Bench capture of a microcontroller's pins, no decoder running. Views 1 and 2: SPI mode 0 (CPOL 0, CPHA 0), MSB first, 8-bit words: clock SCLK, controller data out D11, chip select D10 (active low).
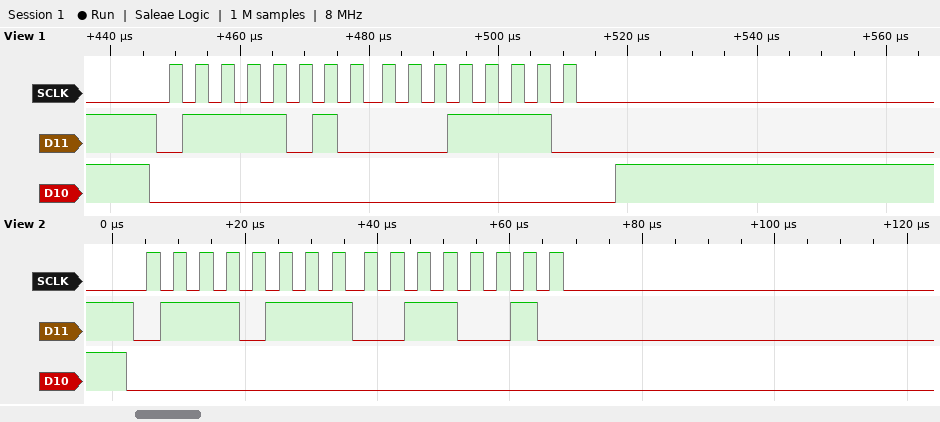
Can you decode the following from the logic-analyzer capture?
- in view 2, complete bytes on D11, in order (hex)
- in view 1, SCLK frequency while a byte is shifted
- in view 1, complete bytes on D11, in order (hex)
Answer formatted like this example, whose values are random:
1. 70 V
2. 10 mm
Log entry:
1. 77 32
2. 250 kHz
3. 7A 1E
